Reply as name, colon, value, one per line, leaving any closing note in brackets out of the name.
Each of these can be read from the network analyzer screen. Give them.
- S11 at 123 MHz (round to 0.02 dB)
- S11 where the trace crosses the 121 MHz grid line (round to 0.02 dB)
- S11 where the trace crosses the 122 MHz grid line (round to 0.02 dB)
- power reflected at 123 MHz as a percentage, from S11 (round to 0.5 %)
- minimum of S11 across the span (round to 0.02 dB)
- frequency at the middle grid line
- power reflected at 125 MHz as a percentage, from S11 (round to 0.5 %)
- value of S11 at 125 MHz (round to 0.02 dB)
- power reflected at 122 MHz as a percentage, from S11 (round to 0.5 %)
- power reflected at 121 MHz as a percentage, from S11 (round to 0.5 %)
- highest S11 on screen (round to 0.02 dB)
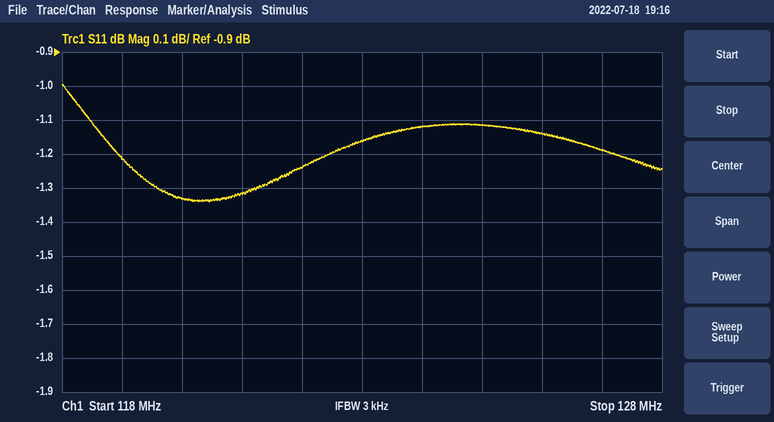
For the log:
S11 at 123 MHz: -1.16 dB
S11 where the trace crosses the 121 MHz grid line: -1.32 dB
S11 where the trace crosses the 122 MHz grid line: -1.24 dB
power reflected at 123 MHz as a percentage, from S11: 76.5 %
minimum of S11 across the span: -1.34 dB
frequency at the middle grid line: 123 MHz
power reflected at 125 MHz as a percentage, from S11: 77.5 %
value of S11 at 125 MHz: -1.12 dB
power reflected at 122 MHz as a percentage, from S11: 75.0 %
power reflected at 121 MHz as a percentage, from S11: 74.0 %
highest S11 on screen: -1.00 dB
